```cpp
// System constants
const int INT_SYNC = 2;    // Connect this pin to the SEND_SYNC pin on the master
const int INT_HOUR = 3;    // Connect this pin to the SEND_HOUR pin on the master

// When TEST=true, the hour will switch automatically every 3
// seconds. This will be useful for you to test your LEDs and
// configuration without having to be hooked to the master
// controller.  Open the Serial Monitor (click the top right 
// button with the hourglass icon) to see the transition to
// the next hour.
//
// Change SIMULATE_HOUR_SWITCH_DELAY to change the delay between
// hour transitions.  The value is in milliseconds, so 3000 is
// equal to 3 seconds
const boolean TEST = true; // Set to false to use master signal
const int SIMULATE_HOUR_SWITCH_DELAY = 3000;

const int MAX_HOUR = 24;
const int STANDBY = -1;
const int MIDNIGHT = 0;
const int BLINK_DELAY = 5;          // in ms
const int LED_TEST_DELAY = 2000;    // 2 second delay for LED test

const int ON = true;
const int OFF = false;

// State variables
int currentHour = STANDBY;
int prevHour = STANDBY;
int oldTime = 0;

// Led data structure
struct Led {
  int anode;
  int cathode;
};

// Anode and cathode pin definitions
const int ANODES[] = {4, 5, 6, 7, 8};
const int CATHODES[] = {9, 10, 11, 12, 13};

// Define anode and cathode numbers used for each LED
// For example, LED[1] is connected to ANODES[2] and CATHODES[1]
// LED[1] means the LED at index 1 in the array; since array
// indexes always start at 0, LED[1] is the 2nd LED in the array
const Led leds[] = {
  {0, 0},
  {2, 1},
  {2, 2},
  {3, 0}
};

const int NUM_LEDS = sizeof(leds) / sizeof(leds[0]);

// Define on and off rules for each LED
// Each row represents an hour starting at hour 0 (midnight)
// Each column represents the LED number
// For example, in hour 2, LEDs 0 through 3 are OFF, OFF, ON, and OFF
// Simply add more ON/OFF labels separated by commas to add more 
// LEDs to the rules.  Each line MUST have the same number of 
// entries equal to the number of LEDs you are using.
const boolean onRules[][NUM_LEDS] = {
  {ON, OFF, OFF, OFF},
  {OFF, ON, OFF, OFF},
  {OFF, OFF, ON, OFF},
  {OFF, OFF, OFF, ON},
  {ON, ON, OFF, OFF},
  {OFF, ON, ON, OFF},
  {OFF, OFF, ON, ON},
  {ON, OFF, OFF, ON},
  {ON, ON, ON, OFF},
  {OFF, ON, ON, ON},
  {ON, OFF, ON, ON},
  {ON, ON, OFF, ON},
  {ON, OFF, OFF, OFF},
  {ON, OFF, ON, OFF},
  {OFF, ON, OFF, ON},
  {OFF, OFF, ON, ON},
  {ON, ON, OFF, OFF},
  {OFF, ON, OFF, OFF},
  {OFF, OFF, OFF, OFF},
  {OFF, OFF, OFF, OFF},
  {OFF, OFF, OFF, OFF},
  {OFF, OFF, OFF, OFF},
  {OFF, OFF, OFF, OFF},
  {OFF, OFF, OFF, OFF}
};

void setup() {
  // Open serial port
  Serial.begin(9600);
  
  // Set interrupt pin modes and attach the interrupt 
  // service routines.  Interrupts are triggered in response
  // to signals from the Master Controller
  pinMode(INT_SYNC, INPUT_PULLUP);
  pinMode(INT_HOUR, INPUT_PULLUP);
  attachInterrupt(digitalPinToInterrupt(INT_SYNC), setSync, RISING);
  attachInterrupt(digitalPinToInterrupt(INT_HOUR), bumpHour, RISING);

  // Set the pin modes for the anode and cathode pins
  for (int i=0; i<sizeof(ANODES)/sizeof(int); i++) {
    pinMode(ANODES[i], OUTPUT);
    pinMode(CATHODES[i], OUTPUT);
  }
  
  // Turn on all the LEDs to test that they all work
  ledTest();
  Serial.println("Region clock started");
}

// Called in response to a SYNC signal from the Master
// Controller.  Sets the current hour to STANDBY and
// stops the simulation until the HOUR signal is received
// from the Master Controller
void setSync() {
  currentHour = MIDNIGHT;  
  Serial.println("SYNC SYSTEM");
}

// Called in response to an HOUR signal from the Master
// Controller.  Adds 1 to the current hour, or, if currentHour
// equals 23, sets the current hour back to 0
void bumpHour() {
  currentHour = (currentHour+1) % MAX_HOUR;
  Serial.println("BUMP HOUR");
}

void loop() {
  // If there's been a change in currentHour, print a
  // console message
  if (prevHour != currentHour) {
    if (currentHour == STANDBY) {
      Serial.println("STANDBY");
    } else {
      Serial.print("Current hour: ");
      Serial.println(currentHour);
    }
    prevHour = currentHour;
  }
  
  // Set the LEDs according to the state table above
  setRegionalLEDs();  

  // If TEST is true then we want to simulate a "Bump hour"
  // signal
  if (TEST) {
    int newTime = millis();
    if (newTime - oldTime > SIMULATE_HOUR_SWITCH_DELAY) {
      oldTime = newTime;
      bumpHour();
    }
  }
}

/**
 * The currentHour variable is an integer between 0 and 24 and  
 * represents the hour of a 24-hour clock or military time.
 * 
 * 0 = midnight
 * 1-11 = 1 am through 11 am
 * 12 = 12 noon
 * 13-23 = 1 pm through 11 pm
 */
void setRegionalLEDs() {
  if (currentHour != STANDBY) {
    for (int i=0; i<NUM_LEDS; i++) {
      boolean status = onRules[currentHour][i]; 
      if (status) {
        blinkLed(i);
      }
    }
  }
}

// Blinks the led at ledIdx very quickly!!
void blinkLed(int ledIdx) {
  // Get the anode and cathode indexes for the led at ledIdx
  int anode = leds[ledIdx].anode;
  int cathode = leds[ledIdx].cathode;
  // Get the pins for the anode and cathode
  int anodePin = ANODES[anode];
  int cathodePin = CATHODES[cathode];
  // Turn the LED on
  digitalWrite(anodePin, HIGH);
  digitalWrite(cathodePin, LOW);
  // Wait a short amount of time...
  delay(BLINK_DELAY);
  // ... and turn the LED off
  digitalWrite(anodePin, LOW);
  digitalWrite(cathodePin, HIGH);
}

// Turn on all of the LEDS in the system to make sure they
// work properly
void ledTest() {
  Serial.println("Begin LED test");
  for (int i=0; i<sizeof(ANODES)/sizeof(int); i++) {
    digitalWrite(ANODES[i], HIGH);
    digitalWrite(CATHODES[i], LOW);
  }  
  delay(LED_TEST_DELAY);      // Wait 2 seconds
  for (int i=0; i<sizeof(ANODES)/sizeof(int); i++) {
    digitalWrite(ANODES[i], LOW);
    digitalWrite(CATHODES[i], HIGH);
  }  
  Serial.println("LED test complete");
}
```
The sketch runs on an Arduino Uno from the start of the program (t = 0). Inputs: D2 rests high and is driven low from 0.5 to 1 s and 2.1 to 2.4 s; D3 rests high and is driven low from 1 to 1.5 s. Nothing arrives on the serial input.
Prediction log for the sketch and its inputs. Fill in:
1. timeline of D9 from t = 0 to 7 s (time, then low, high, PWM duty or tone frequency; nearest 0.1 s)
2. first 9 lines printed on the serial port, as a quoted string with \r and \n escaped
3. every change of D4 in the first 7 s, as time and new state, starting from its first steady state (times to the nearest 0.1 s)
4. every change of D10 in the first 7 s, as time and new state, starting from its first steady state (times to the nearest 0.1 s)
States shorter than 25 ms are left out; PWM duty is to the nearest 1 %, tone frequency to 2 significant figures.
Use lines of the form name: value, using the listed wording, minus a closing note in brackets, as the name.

timeline of D9 from t = 0 to 7 s: 0 s low; 2 s high; 2.4 s tone 200 Hz; 3 s high
first 9 lines printed on the serial port, as a quoted string with \r and \n escaped: "Begin LED test\r\nSYNC SYSTEM\r\nBUMP HOUR\r\nLED test complete\r\nRegion clock started\r\nCurrent hour: 1\r\nSYNC SYSTEM\r\nCurrent hour: 0\r\nBUMP HOUR\r\n"
every change of D4 in the first 7 s, as time and new state, starting from its first steady state: 0 s high; 2 s low; 2.4 s tone 200 Hz; 3 s low
every change of D10 in the first 7 s, as time and new state, starting from its first steady state: 0 s low; 2 s tone 200 Hz; 2.4 s high; 3 s tone 200 Hz; 6 s high
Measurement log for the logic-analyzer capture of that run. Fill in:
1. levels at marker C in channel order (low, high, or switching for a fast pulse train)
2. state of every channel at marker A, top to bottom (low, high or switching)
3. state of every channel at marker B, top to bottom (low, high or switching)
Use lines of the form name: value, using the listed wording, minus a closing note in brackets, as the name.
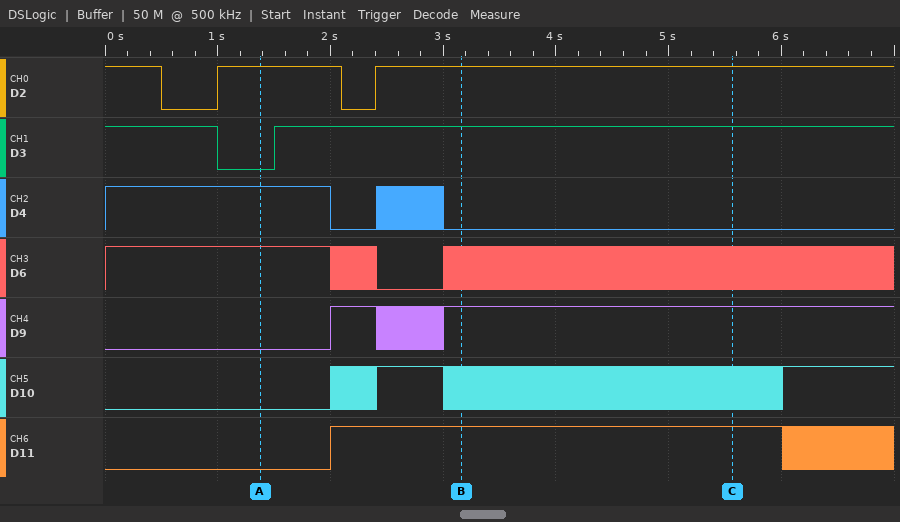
levels at marker C in channel order: D2 high, D3 high, D4 low, D6 switching, D9 high, D10 switching, D11 high
state of every channel at marker A, top to bottom: D2 high, D3 low, D4 high, D6 high, D9 low, D10 low, D11 low
state of every channel at marker B, top to bottom: D2 high, D3 high, D4 low, D6 switching, D9 high, D10 switching, D11 high
